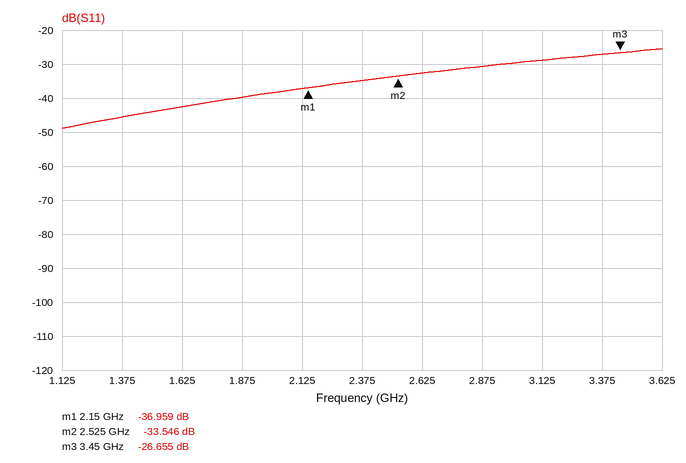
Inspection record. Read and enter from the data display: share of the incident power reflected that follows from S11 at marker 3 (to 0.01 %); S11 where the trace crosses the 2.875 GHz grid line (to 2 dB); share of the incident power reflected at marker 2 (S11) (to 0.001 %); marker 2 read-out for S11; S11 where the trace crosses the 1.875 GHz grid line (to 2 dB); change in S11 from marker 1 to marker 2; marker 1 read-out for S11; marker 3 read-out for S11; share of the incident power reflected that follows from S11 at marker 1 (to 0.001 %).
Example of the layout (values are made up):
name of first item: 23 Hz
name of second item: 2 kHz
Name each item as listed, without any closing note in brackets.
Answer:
share of the incident power reflected that follows from S11 at marker 3: 0.22 %
S11 where the trace crosses the 2.875 GHz grid line: -30 dB
share of the incident power reflected at marker 2 (S11): 0.044 %
marker 2 read-out for S11: -33.546 dB
S11 where the trace crosses the 1.875 GHz grid line: -40 dB
change in S11 from marker 1 to marker 2: 3.413 dB
marker 1 read-out for S11: -36.959 dB
marker 3 read-out for S11: -26.655 dB
share of the incident power reflected that follows from S11 at marker 1: 0.020 %
